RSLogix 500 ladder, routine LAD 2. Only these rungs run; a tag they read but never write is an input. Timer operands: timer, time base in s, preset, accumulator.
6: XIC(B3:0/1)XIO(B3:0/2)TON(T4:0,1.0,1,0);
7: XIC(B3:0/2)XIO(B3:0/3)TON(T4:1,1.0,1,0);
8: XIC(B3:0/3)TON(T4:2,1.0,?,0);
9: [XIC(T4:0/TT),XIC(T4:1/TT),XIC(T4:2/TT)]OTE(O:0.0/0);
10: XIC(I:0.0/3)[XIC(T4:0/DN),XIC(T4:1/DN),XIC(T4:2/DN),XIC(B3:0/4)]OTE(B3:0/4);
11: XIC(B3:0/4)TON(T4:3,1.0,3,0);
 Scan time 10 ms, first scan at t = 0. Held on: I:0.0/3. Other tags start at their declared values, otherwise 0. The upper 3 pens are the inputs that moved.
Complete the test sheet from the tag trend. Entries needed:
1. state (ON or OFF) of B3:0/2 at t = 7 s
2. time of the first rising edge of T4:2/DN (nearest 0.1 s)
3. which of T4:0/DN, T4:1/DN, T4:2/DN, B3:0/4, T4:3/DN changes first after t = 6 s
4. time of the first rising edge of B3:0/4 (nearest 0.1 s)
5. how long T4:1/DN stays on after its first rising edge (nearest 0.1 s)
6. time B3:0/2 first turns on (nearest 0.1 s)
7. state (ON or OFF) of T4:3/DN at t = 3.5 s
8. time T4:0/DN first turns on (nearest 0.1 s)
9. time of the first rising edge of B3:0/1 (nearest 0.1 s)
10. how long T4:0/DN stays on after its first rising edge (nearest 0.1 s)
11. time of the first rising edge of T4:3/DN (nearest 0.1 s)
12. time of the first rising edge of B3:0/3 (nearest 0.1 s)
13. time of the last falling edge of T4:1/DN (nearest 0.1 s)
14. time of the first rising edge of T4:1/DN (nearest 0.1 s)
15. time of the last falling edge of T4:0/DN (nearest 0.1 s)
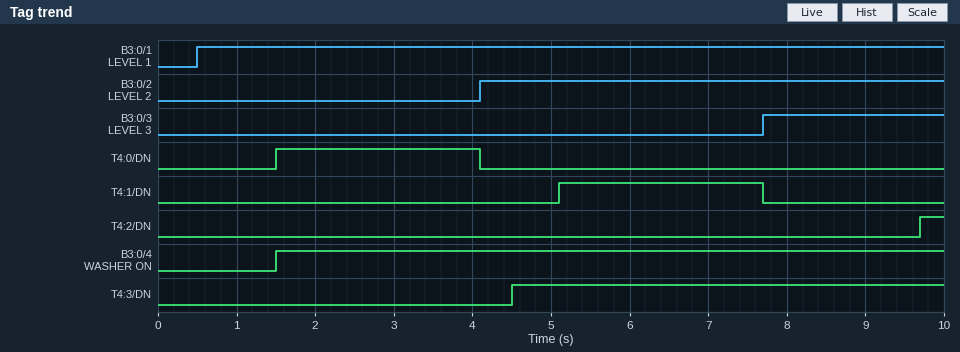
ON
9.7 s
T4:1/DN
1.5 s
2.6 s
4.1 s
OFF
1.5 s
0.5 s
2.6 s
4.5 s
7.7 s
7.7 s
5.1 s
4.1 s
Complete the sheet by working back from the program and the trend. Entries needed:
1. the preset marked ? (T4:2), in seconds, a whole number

2 s
